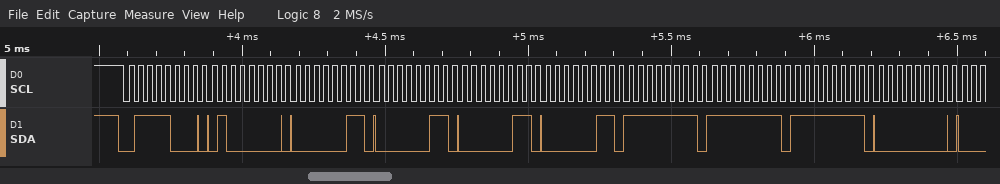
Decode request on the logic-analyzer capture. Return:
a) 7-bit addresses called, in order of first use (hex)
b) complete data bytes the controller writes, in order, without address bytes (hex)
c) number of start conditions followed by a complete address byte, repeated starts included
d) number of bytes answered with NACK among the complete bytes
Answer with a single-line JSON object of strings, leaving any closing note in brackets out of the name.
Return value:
{"7-bit addresses called, in order of first use": "0x3C", "complete data bytes the controller writes, in order, without address bytes": "40 03 03 03 03 FF FF FF 00", "number of start conditions followed by a complete address byte, repeated starts included": "1", "number of bytes answered with NACK among the complete bytes": "0"}
